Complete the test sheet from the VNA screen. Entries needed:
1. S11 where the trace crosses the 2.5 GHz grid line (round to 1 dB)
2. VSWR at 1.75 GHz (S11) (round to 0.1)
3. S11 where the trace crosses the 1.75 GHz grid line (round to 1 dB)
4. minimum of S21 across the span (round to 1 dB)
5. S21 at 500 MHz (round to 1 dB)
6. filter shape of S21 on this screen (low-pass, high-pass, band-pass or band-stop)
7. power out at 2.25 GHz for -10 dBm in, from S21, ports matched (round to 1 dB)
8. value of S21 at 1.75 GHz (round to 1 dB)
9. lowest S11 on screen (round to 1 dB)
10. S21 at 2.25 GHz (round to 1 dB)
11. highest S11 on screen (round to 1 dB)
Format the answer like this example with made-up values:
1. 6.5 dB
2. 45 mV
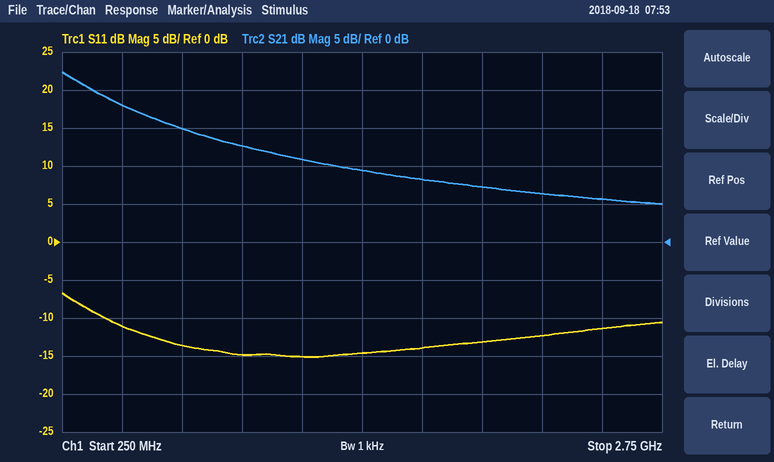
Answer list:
1. -11 dB
2. 1.5
3. -14 dB
4. 5 dB
5. 18 dB
6. low-pass
7. -4 dBm
8. 8 dB
9. -15 dB
10. 6 dB
11. -7 dB
